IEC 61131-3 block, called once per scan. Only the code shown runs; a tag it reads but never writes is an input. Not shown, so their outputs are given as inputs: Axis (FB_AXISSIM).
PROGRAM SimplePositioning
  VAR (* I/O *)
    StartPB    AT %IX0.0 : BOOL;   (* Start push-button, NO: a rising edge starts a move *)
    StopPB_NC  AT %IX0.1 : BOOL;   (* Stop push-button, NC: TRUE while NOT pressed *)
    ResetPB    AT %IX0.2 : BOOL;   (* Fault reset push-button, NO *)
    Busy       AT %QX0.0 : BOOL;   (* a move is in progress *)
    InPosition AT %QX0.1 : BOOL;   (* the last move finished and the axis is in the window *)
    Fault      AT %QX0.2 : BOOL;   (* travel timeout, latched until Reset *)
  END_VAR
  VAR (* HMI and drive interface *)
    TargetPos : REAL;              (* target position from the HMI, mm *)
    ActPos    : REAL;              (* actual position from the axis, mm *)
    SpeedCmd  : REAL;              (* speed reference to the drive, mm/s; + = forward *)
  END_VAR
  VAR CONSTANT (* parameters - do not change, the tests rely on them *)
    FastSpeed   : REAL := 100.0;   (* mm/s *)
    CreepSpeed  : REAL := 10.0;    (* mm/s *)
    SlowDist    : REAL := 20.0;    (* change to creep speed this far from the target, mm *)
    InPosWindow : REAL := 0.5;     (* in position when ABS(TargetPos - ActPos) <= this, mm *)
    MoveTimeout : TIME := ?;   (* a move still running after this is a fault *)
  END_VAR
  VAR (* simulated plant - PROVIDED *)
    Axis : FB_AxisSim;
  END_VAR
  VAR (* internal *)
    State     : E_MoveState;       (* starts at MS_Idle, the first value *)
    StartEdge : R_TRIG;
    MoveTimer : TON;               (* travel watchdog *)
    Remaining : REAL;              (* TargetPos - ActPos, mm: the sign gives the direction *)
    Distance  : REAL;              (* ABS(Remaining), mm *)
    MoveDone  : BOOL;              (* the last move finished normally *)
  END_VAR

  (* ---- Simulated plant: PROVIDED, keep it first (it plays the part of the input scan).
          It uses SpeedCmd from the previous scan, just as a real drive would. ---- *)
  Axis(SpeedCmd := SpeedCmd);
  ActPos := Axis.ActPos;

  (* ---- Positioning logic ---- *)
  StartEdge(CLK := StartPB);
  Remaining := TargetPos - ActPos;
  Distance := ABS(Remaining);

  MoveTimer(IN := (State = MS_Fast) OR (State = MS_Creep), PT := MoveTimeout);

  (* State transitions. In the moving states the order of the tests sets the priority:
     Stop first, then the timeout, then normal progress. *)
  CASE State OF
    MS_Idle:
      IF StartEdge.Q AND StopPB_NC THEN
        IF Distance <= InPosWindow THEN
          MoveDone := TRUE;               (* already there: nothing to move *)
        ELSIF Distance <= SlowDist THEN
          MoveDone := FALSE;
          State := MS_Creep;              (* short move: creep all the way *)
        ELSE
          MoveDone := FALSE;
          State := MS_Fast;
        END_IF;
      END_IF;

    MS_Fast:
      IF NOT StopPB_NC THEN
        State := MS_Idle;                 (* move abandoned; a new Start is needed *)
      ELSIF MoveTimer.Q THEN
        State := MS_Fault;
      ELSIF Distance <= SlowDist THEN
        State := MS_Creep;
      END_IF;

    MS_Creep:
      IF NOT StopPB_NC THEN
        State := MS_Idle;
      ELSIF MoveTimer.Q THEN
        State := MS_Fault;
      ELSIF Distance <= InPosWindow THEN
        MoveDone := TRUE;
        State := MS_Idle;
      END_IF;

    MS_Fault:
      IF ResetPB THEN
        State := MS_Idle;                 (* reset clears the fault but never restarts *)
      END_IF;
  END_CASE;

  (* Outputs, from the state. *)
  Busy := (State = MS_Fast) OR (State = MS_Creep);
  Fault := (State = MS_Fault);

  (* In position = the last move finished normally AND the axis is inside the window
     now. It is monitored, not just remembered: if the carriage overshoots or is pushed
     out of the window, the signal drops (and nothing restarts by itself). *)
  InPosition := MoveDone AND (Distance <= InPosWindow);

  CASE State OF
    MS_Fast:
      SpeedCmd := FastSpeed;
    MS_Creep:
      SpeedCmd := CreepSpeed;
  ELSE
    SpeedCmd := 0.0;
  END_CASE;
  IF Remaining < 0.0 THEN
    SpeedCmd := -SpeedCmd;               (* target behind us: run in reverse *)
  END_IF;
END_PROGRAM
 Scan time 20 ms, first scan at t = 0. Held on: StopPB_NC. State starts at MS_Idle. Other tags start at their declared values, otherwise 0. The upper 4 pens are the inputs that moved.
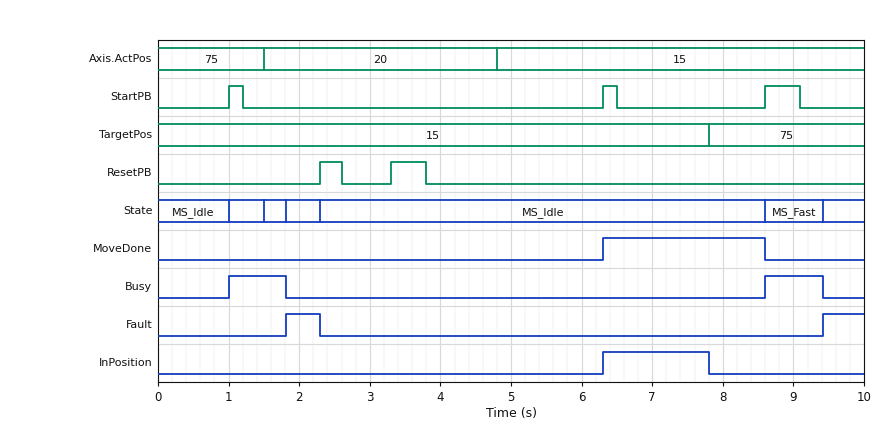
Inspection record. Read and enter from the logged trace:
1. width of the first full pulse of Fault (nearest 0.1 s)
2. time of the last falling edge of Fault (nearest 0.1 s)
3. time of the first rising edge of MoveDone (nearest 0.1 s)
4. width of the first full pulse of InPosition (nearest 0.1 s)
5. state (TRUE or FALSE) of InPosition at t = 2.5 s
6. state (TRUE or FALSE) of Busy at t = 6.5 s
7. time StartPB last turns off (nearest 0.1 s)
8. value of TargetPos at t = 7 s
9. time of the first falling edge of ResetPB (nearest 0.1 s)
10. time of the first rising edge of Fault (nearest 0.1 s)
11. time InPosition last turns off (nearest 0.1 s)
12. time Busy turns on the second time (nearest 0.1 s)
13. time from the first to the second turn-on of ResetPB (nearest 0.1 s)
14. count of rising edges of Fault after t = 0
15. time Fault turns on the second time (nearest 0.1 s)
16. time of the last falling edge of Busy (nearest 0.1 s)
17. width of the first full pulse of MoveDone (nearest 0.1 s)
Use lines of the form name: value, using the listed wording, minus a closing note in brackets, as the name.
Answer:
width of the first full pulse of Fault: 0.5 s
time of the last falling edge of Fault: 2.3 s
time of the first rising edge of MoveDone: 6.3 s
width of the first full pulse of InPosition: 1.5 s
state (TRUE or FALSE) of InPosition at t = 2.5 s: FALSE
state (TRUE or FALSE) of Busy at t = 6.5 s: FALSE
time StartPB last turns off: 9.1 s
value of TargetPos at t = 7 s: 15
time of the first falling edge of ResetPB: 2.6 s
time of the first rising edge of Fault: 1.8 s
time InPosition last turns off: 7.8 s
time Busy turns on the second time: 8.6 s
time from the first to the second turn-on of ResetPB: 1.0 s
count of rising edges of Fault after t = 0: 2
time Fault turns on the second time: 9.4 s
time of the last falling edge of Busy: 9.4 s
width of the first full pulse of MoveDone: 2.3 s
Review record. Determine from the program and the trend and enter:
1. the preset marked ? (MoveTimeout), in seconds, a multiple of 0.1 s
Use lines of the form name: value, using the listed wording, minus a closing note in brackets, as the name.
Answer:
the preset marked ? (MoveTimeout), in seconds, a multiple of 0.1 s: 0.8 s
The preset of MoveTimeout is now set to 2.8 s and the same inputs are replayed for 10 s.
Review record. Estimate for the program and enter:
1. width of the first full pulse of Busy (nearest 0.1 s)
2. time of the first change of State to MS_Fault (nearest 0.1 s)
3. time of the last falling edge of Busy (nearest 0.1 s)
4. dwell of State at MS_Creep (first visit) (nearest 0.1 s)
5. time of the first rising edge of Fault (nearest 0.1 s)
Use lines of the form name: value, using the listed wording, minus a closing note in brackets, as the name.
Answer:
width of the first full pulse of Busy: 2.8 s
time of the first change of State to MS_Fault: 3.8 s
time of the last falling edge of Busy: 3.8 s
dwell of State at MS_Creep (first visit): 2.3 s
time of the first rising edge of Fault: 3.8 s
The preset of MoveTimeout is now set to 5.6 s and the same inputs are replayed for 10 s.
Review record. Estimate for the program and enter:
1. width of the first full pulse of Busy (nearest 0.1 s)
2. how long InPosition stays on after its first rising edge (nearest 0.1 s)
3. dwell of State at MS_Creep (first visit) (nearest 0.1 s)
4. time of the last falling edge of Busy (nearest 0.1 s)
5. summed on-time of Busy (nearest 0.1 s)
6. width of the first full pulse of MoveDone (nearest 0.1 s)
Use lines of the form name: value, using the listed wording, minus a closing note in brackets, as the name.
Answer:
width of the first full pulse of Busy: 3.8 s
how long InPosition stays on after its first rising edge: 3.0 s
dwell of State at MS_Creep (first visit): 3.3 s
time of the last falling edge of Busy: 4.8 s
summed on-time of Busy: 5.2 s
width of the first full pulse of MoveDone: 3.8 s
